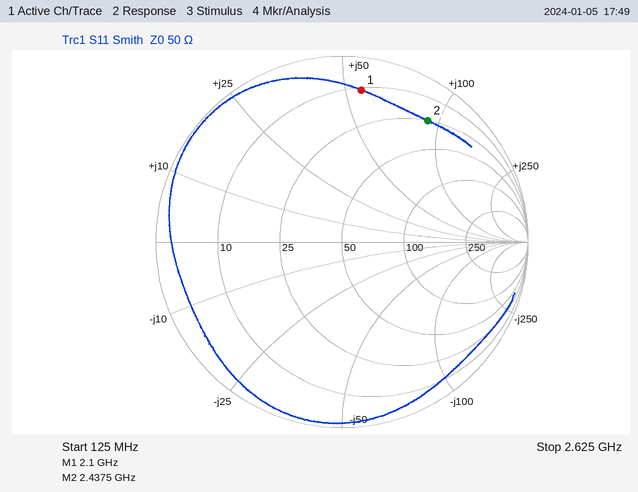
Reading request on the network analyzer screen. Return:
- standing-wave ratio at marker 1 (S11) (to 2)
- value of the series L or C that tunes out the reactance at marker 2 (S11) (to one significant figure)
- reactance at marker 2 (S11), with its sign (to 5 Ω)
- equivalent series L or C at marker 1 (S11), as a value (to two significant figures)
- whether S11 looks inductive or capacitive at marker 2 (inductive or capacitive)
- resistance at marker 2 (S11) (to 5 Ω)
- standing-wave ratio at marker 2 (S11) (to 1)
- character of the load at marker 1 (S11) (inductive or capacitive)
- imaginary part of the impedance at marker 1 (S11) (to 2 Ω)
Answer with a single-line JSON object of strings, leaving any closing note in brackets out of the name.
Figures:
{"standing-wave ratio at marker 1 (S11)": "10", "value of the series L or C that tunes out the reactance at marker 2 (S11)": "700 fF", "reactance at marker 2 (S11), with its sign": "+90 Ω", "equivalent series L or C at marker 1 (S11), as a value": "4.2 nH", "whether S11 looks inductive or capacitive at marker 2": "inductive", "resistance at marker 2 (S11)": "25 Ω", "standing-wave ratio at marker 2 (S11)": "9", "character of the load at marker 1 (S11)": "inductive", "imaginary part of the impedance at marker 1 (S11)": "+56 Ω"}
